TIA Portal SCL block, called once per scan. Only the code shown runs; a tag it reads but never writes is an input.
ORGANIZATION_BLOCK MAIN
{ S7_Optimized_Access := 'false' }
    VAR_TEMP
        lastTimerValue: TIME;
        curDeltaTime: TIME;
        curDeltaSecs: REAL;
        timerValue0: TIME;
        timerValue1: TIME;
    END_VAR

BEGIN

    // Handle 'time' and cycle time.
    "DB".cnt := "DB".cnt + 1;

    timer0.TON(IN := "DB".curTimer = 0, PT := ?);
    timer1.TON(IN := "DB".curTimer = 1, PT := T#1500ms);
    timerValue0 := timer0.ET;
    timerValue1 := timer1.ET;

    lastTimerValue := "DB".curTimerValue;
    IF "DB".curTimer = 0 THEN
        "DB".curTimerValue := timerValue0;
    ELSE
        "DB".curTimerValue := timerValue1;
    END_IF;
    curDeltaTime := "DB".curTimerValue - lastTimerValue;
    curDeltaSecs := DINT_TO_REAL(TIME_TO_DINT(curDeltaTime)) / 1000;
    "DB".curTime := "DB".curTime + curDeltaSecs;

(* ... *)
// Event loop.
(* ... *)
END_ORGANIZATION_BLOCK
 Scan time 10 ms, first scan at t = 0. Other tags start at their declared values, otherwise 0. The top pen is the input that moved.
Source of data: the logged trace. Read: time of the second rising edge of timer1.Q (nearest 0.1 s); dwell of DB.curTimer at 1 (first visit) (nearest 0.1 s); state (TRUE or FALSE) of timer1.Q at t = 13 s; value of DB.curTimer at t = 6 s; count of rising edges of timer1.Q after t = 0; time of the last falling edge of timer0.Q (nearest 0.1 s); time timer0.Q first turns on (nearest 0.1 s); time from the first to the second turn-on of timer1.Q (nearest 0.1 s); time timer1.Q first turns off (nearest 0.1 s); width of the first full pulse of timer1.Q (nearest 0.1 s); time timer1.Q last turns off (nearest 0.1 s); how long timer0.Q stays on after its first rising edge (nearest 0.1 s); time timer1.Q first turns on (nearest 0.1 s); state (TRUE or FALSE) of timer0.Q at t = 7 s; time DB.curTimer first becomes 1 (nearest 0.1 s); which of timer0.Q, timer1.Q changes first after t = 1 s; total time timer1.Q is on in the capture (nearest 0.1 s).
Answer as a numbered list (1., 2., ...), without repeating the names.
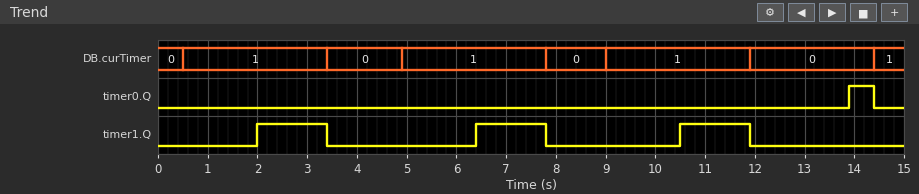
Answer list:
1. 6.4 s
2. 2.9 s
3. FALSE
4. 1
5. 3
6. 14.4 s
7. 13.9 s
8. 4.4 s
9. 3.4 s
10. 1.4 s
11. 11.9 s
12. 0.5 s
13. 2.0 s
14. FALSE
15. 0.5 s
16. timer1.Q
17. 4.2 s
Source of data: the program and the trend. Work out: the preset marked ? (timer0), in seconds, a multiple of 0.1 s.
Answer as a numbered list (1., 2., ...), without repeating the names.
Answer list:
1. 2.0 s
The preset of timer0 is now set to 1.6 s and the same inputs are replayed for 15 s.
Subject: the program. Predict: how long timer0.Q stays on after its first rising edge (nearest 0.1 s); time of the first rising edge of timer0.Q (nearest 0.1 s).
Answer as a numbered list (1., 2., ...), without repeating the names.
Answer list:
1. 0.9 s
2. 13.5 s
